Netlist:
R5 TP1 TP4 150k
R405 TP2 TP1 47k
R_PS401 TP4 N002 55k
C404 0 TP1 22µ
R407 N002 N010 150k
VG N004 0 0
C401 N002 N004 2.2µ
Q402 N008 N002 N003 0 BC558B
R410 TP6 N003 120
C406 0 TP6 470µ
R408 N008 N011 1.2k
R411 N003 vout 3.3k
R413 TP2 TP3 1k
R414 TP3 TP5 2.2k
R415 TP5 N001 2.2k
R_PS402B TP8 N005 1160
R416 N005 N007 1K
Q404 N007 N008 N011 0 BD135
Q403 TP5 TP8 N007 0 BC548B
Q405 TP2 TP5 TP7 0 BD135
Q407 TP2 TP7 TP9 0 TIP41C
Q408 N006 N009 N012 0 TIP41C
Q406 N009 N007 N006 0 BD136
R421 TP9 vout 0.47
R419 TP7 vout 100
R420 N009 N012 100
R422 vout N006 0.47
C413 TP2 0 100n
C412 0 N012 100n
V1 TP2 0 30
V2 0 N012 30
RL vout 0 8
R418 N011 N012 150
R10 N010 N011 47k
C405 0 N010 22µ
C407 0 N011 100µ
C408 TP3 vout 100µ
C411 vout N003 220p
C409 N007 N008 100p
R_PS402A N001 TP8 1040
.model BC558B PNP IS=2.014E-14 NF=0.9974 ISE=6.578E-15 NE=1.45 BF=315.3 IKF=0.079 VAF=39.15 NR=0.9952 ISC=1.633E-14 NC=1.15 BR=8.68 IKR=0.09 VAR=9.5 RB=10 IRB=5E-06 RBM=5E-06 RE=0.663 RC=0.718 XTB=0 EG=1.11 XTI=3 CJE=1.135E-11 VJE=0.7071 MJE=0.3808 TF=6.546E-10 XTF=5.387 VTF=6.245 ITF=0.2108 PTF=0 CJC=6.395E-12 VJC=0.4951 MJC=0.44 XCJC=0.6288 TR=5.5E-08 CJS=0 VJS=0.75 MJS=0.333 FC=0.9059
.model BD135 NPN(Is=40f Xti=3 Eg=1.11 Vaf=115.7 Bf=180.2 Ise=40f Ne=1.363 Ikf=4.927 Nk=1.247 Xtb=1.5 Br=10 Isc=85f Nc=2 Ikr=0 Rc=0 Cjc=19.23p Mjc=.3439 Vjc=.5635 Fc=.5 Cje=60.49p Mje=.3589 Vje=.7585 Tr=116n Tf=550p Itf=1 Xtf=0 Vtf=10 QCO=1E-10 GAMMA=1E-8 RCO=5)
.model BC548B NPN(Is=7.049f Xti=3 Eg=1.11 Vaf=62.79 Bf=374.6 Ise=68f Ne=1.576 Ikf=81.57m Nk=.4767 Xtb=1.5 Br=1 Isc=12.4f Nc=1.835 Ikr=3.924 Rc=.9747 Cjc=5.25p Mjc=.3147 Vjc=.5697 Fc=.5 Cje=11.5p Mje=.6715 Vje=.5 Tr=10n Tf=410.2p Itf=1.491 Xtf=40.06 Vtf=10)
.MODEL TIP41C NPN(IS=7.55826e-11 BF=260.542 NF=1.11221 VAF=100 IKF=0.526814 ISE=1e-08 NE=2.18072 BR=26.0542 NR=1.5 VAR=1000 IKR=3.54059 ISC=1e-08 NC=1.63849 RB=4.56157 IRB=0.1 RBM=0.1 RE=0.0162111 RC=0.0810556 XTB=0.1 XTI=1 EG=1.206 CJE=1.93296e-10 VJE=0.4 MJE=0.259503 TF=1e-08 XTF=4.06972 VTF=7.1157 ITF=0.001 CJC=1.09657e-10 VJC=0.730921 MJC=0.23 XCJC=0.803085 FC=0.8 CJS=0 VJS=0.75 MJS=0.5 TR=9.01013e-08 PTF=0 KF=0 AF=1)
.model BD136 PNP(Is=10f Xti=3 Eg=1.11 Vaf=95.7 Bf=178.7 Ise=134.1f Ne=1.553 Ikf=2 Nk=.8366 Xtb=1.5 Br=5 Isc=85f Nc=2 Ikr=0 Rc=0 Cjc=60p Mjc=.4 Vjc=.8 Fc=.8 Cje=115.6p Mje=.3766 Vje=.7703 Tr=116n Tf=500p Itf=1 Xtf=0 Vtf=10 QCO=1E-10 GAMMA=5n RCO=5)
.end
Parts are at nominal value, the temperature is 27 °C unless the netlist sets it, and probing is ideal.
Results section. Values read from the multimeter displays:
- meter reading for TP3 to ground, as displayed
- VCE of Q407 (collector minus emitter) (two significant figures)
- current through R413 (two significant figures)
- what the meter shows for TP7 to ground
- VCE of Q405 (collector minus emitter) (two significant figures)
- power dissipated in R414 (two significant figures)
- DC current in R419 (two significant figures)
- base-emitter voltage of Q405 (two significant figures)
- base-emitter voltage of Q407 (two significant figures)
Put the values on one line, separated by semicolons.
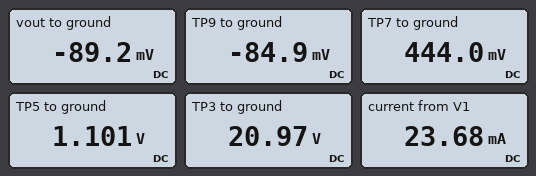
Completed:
20.97 V; 30 V; 9.0 mA; 444.0 mV; 30 V; 180 mW; 5.3 mA; 660 mV; 530 mV
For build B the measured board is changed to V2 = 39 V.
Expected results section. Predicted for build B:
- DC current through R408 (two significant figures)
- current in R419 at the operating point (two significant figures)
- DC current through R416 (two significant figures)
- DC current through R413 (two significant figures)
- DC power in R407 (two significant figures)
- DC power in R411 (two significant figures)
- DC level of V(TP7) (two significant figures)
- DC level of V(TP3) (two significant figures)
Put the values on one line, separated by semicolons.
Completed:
560 µA; 2.8 mA; 340 µA; 11 mA; 3.4 mW; 1.3 mW; -4.7 V; 19 V
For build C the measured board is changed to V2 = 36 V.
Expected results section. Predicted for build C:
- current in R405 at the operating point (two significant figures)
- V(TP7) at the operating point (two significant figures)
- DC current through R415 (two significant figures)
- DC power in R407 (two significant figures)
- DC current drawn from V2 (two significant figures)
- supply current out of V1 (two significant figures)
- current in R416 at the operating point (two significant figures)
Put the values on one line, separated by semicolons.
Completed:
140 µA; -3.0 V; 370 µA; 3.1 mW; 430 mA; 14 mA; 340 µA
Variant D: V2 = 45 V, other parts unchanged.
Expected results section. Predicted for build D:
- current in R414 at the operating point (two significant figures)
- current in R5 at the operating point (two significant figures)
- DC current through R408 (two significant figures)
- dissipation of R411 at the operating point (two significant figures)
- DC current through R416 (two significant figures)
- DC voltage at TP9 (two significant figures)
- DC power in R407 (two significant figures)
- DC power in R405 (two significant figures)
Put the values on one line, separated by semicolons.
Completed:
12 mA; 160 µA; 560 µA; 1.3 mW; 340 µA; -8.2 V; 4.0 mW; 1.2 mW
